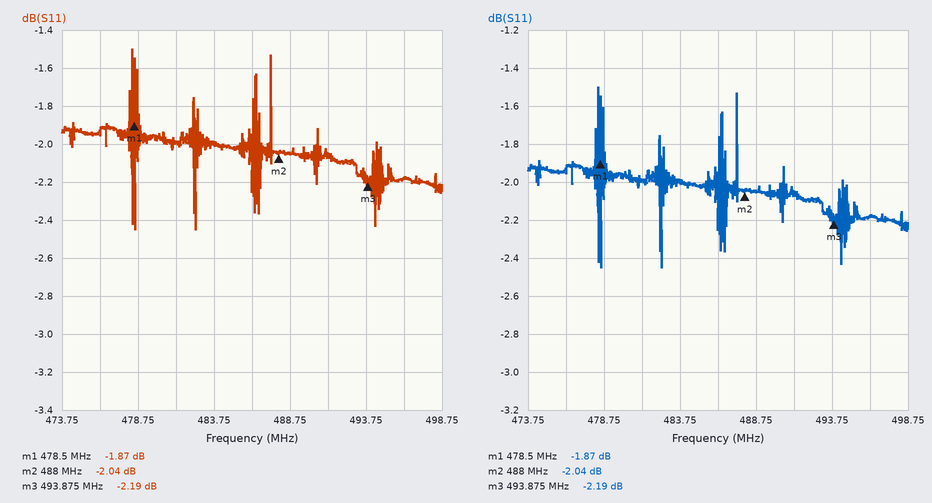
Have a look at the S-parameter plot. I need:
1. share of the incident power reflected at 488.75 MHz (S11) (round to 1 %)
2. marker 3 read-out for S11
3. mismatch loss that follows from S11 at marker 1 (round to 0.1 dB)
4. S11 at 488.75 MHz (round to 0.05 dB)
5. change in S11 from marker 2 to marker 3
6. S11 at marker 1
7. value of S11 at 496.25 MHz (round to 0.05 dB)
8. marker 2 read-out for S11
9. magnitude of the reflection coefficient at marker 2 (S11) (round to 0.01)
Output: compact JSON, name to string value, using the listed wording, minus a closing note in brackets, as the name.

{"share of the incident power reflected at 488.75 MHz (S11)": "62 %", "marker 3 read-out for S11": "-2.19 dB", "mismatch loss that follows from S11 at marker 1": "4.6 dB", "S11 at 488.75 MHz": "-2.05 dB", "change in S11 from marker 2 to marker 3": "-0.15 dB", "S11 at marker 1": "-1.87 dB", "value of S11 at 496.25 MHz": "-2.20 dB", "marker 2 read-out for S11": "-2.04 dB", "magnitude of the reflection coefficient at marker 2 (S11)": "0.79"}
